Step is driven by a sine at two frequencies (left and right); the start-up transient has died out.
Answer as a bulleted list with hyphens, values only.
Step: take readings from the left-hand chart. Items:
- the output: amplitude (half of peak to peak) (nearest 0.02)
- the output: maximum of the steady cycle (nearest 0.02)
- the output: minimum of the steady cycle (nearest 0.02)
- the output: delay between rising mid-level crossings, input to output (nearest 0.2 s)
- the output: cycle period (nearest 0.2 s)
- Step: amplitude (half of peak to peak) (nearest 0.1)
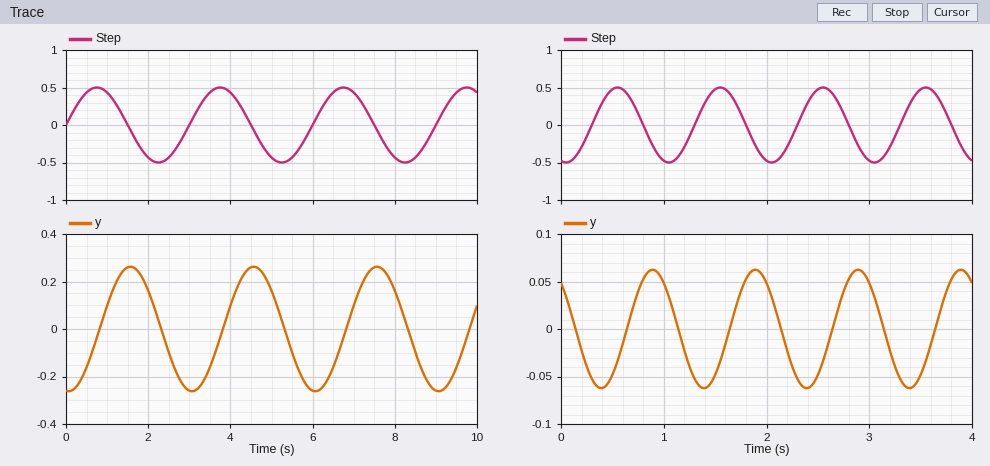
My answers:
- 0.26
- 0.26
- -0.26
- 0.8 s
- 3.0 s
- 0.5
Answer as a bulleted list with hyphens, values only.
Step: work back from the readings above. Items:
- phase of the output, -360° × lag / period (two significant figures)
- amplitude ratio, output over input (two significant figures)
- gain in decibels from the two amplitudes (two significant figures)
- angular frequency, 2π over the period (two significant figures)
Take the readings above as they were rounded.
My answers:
- -96°
- 0.52
- -5.7 dB
- 2.1 rad/s
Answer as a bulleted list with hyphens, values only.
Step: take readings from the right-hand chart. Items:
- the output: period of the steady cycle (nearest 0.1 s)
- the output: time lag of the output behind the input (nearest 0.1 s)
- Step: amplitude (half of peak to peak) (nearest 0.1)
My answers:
- 1.0 s
- 0.3 s
- 0.5
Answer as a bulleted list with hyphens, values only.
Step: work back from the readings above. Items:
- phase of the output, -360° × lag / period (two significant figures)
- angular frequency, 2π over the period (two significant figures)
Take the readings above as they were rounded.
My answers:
- -110°
- 6.3 rad/s
